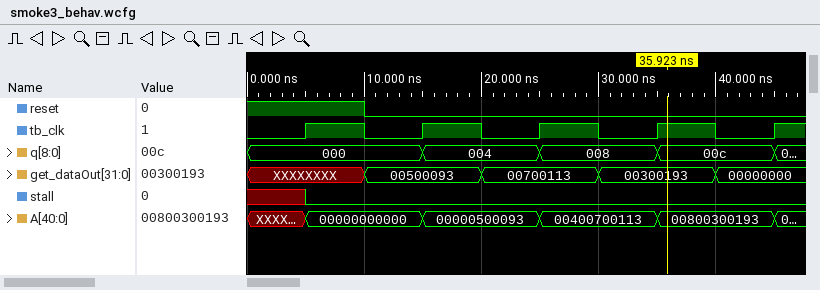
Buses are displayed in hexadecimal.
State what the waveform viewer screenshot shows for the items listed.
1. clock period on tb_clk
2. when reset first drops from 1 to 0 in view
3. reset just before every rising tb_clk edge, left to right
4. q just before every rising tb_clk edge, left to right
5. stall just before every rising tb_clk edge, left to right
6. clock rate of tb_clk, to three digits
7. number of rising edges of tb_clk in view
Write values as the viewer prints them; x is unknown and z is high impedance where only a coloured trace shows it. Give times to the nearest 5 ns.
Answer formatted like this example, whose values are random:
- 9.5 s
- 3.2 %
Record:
- 10 ns
- 10 ns
- 1 0 0 0 0
- 000, 000, 004, 008, 00c
- x 0 0 0 0
- 100 MHz
- 5
